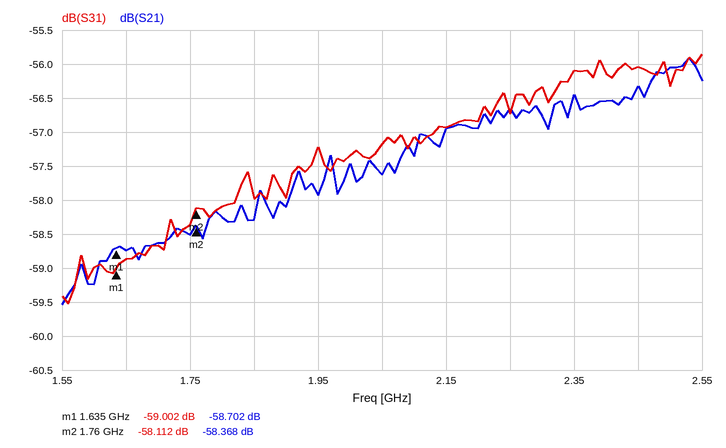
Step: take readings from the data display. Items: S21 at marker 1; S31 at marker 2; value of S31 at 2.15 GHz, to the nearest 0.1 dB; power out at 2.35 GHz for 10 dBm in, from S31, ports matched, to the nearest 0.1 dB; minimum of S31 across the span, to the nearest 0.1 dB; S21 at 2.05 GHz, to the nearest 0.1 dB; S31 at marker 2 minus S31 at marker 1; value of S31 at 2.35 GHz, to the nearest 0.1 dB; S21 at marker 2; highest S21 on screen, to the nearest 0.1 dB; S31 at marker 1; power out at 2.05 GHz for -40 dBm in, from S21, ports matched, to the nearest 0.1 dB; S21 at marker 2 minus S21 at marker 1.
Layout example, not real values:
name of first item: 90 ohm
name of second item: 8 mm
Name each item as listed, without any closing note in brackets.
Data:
S21 at marker 1: -58.702 dB
S31 at marker 2: -58.112 dB
value of S31 at 2.15 GHz, to the nearest 0.1 dB: -56.9 dB
power out at 2.35 GHz for 10 dBm in, from S31, ports matched, to the nearest 0.1 dB: -46.1 dBm
minimum of S31 across the span, to the nearest 0.1 dB: -59.5 dB
S21 at 2.05 GHz, to the nearest 0.1 dB: -57.6 dB
S31 at marker 2 minus S31 at marker 1: 0.890 dB
value of S31 at 2.35 GHz, to the nearest 0.1 dB: -56.1 dB
S21 at marker 2: -58.368 dB
highest S21 on screen, to the nearest 0.1 dB: -55.9 dB
S31 at marker 1: -59.002 dB
power out at 2.05 GHz for -40 dBm in, from S21, ports matched, to the nearest 0.1 dB: -97.6 dBm
S21 at marker 2 minus S21 at marker 1: 0.334 dB
